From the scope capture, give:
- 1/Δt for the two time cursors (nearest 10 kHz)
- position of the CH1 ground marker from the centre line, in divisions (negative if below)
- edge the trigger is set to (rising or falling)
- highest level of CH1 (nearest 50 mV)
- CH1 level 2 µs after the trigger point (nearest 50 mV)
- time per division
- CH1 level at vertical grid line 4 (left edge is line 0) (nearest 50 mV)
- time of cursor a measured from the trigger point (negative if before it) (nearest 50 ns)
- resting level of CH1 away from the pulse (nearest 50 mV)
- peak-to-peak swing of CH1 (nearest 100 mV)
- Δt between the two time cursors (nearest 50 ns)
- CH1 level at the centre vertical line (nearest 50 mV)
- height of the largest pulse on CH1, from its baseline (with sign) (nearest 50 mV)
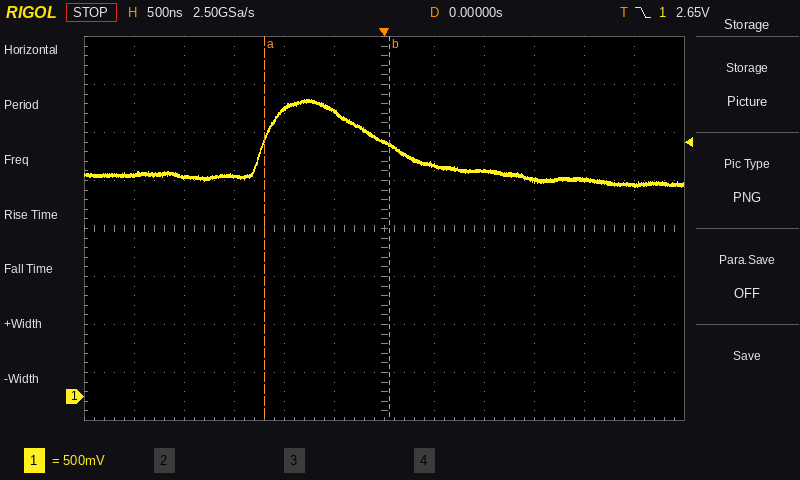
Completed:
800 kHz
-3.5 div
falling
3.10 V
2.25 V
500 ns
3.00 V
-1.20 µs
2.30 V
900 mV
1.25 µs
2.65 V
+800 mV
